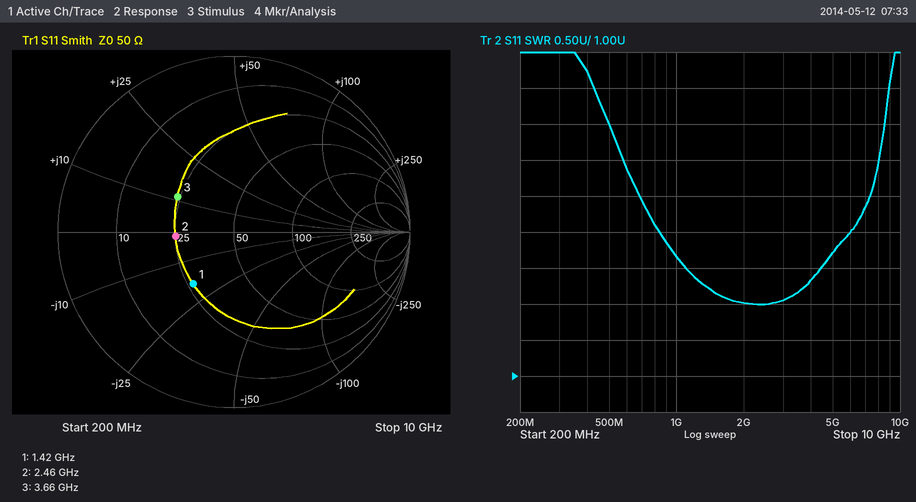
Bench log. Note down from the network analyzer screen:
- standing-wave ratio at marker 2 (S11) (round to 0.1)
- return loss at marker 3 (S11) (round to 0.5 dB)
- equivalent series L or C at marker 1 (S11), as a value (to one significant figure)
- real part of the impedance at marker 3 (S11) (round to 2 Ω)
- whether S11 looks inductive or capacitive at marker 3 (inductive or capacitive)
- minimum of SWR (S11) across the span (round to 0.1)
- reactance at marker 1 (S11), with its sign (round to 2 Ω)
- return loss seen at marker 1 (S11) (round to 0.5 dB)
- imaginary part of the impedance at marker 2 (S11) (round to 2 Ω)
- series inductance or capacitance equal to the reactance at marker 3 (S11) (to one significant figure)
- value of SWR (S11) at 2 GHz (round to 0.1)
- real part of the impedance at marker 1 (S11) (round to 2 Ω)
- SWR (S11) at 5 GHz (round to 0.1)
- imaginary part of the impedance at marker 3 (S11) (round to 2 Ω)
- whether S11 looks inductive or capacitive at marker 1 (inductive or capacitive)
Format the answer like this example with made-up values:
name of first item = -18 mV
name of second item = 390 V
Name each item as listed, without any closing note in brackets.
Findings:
standing-wave ratio at marker 2 (S11) = 2.0
return loss at marker 3 (S11) = 8.5 dB
equivalent series L or C at marker 1 (S11), as a value = 6 pF
real part of the impedance at marker 3 (S11) = 24 Ω
whether S11 looks inductive or capacitive at marker 3 = inductive
minimum of SWR (S11) across the span = 2.0
reactance at marker 1 (S11), with its sign = -18 Ω
return loss seen at marker 1 (S11) = 8.5 dB
imaginary part of the impedance at marker 2 (S11) = -2 Ω
series inductance or capacitance equal to the reactance at marker 3 (S11) = 500 pH
value of SWR (S11) at 2 GHz = 2.0
real part of the impedance at marker 1 (S11) = 26 Ω
SWR (S11) at 5 GHz = 2.7
imaginary part of the impedance at marker 3 (S11) = +12 Ω
whether S11 looks inductive or capacitive at marker 1 = capacitive
